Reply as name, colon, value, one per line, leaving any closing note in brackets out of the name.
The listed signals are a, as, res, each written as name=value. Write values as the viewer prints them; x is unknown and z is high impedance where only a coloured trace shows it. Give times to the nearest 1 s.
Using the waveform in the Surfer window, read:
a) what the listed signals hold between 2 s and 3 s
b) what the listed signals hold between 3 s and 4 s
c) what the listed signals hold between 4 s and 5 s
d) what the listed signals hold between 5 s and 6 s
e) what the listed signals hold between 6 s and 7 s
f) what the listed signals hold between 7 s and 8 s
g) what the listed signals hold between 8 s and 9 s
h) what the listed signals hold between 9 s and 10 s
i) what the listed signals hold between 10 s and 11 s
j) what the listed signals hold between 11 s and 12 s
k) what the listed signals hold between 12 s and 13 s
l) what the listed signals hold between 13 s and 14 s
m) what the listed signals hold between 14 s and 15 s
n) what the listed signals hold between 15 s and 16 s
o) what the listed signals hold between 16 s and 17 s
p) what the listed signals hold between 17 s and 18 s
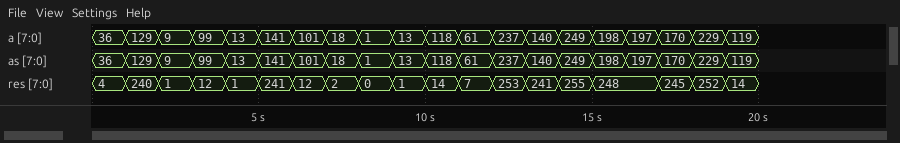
what the listed signals hold between 2 s and 3 s: a=9, as=9, res=1
what the listed signals hold between 3 s and 4 s: a=99, as=99, res=12
what the listed signals hold between 4 s and 5 s: a=13, as=13, res=1
what the listed signals hold between 5 s and 6 s: a=141, as=141, res=241
what the listed signals hold between 6 s and 7 s: a=101, as=101, res=12
what the listed signals hold between 7 s and 8 s: a=18, as=18, res=2
what the listed signals hold between 8 s and 9 s: a=1, as=1, res=0
what the listed signals hold between 9 s and 10 s: a=13, as=13, res=1
what the listed signals hold between 10 s and 11 s: a=118, as=118, res=14
what the listed signals hold between 11 s and 12 s: a=61, as=61, res=7
what the listed signals hold between 12 s and 13 s: a=237, as=237, res=253
what the listed signals hold between 13 s and 14 s: a=140, as=140, res=241
what the listed signals hold between 14 s and 15 s: a=249, as=249, res=255
what the listed signals hold between 15 s and 16 s: a=198, as=198, res=248
what the listed signals hold between 16 s and 17 s: a=197, as=197, res=248
what the listed signals hold between 17 s and 18 s: a=170, as=170, res=245
